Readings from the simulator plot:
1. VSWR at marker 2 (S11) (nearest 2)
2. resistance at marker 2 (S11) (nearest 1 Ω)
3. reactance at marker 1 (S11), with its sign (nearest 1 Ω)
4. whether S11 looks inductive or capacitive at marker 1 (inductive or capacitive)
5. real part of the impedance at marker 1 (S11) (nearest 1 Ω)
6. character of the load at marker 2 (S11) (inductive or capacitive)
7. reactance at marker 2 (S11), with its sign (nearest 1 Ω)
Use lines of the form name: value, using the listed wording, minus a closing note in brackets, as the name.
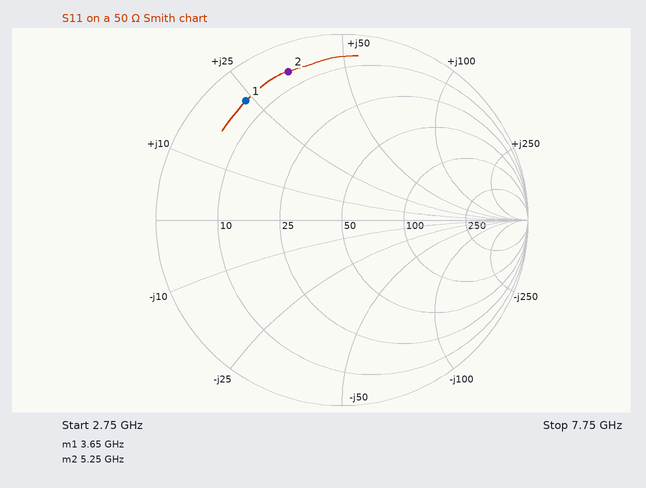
VSWR at marker 2 (S11): 12
resistance at marker 2 (S11): 6 Ω
reactance at marker 1 (S11), with its sign: +24 Ω
whether S11 looks inductive or capacitive at marker 1: inductive
real part of the impedance at marker 1 (S11): 6 Ω
character of the load at marker 2 (S11): inductive
reactance at marker 2 (S11), with its sign: +35 Ω
